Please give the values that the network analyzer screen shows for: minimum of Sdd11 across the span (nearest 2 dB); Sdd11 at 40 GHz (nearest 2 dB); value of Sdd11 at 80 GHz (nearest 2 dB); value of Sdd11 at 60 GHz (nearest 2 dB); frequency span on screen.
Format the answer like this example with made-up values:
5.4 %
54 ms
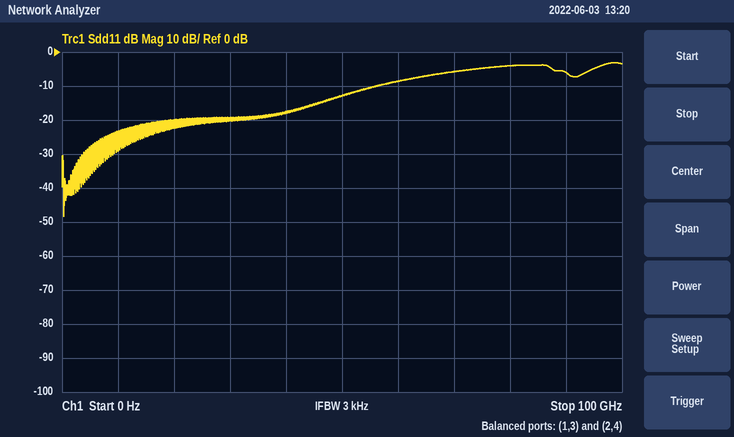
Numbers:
-48 dB
-18 dB
-4 dB
-8 dB
100 GHz
